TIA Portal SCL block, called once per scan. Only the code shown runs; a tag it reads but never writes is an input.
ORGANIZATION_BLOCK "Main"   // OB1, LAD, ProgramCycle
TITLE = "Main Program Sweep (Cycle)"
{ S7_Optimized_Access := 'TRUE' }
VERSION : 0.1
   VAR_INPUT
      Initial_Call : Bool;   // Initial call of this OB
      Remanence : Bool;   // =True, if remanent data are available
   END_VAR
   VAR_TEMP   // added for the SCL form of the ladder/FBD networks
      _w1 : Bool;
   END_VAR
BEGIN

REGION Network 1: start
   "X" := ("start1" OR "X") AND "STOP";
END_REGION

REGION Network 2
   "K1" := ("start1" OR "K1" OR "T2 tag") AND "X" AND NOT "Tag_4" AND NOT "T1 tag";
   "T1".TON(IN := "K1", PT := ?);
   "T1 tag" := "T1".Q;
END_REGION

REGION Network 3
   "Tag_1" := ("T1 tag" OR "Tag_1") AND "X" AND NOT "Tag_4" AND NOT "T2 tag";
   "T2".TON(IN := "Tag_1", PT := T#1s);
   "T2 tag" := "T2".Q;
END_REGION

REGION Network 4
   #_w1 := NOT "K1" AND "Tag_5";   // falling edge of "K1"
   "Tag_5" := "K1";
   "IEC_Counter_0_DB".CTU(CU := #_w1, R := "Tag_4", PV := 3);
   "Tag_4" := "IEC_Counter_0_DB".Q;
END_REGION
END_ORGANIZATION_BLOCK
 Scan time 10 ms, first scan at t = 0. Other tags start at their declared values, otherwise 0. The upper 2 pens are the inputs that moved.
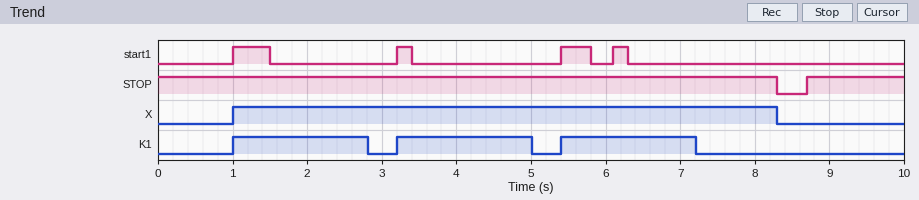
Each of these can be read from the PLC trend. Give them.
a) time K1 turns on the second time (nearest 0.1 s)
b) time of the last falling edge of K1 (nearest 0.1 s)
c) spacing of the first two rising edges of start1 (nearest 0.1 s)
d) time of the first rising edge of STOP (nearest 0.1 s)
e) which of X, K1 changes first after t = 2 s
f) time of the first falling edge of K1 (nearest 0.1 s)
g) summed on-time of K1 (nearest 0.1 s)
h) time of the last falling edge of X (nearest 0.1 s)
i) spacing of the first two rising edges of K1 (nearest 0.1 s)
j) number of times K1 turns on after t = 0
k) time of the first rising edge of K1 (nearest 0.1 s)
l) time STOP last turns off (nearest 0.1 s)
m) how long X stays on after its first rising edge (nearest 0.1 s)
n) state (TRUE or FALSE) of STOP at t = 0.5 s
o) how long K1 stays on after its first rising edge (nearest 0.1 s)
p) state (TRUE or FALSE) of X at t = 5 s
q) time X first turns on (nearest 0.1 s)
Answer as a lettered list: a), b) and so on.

a) 3.2 s
b) 7.2 s
c) 2.2 s
d) 8.7 s
e) K1
f) 2.8 s
g) 5.4 s
h) 8.3 s
i) 2.2 s
j) 3
k) 1.0 s
l) 8.3 s
m) 7.3 s
n) TRUE
o) 1.8 s
p) TRUE
q) 1.0 s
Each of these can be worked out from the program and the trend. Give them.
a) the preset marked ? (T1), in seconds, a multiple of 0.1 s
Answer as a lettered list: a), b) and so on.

a) 1.8 s
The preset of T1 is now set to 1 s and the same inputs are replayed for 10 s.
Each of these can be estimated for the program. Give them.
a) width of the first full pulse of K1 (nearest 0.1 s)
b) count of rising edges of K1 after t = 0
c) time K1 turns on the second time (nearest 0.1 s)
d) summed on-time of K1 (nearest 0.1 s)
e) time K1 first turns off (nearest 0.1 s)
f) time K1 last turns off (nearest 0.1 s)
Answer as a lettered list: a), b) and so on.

a) 1.0 s
b) 5
c) 3.0 s
d) 4.2 s
e) 2.0 s
f) 8.3 s
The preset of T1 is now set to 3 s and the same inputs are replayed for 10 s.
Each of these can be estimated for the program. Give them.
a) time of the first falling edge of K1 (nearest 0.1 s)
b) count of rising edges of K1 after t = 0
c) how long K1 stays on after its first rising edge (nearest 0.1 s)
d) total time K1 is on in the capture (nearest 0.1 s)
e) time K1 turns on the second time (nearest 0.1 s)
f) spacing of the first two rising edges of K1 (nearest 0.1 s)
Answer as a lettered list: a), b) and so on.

a) 4.0 s
b) 2
c) 3.0 s
d) 6.0 s
e) 5.0 s
f) 4.0 s
